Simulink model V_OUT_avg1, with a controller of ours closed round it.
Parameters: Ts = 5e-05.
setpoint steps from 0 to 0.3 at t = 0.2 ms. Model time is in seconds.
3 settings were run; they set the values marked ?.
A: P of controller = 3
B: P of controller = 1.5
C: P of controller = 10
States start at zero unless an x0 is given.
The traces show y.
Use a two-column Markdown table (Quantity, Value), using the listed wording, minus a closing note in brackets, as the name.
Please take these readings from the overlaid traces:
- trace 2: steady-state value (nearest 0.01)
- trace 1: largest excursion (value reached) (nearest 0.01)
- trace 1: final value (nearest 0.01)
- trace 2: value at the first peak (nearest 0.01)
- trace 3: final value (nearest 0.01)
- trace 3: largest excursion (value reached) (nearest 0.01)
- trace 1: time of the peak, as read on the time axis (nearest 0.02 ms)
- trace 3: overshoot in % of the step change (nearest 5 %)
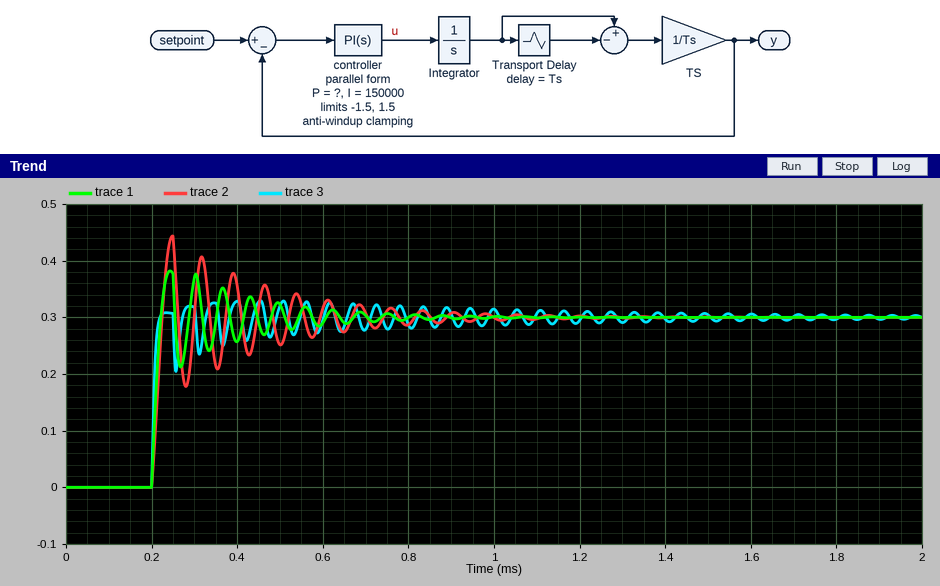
| Quantity | Value |
|---|---|
| trace 2: steady-state value | 0.30 |
| trace 1: largest excursion (value reached) | 0.38 |
| trace 1: final value | 0.30 |
| trace 2: value at the first peak | 0.44 |
| trace 3: final value | 0.30 |
| trace 3: largest excursion (value reached) | 0.33 |
| trace 1: time of the peak, as read on the time axis | 0.24 ms |
| trace 3: overshoot in % of the step change | 10 % |
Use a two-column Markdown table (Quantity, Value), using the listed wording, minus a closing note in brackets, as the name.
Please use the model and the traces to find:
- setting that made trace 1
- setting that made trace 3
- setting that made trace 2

| Quantity | Value |
|---|---|
| setting that made trace 1 | A |
| setting that made trace 3 | C |
| setting that made trace 2 | B |
